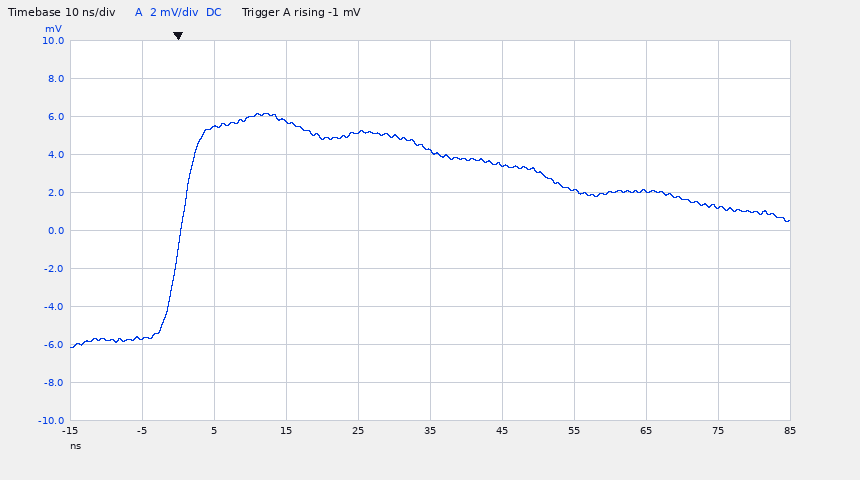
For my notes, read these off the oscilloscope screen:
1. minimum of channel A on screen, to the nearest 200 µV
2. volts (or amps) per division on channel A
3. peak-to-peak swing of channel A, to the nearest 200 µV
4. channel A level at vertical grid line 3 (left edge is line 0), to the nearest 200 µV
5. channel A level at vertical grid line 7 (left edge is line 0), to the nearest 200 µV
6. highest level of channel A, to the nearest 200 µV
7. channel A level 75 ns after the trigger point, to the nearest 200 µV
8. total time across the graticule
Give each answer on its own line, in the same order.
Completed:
-6.2 mV
2 mV
12.4 mV
5.8 mV
2.2 mV
6.2 mV
1.2 mV
100 ns
